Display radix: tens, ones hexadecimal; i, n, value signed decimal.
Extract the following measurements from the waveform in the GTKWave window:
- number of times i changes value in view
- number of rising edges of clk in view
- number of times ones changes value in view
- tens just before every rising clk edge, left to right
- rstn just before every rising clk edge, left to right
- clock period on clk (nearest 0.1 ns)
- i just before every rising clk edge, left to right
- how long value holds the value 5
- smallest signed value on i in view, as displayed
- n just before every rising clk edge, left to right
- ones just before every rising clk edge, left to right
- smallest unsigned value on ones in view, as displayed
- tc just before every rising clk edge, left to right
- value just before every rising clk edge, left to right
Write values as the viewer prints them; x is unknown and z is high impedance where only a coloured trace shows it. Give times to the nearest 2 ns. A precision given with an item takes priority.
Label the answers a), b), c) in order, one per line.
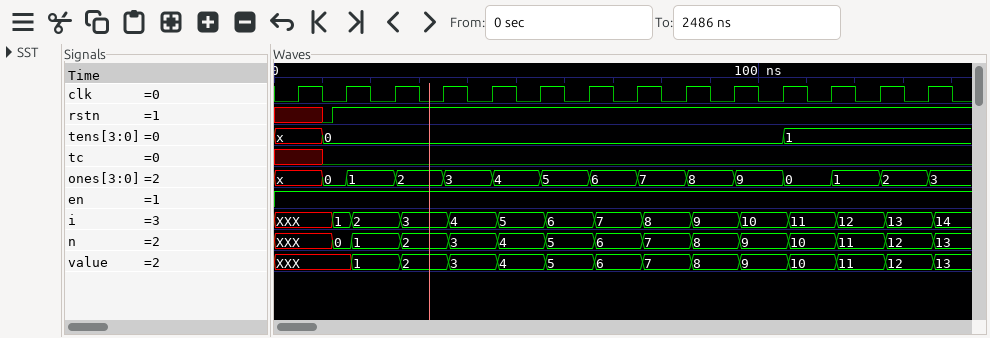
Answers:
a) 14
b) 14
c) 14
d) x, 0, 0, 0, 0, 0, 0, 0, 0, 0, 0, 1, 1, 1
e) x 1 1 1 1 1 1 1 1 1 1 1 1 1
f) 10 ns
g) XXX, 1, 2, 3, 4, 5, 6, 7, 8, 9, 10, 11, 12, 13
h) 10 ns
i) 1
j) XXX, 0, 1, 2, 3, 4, 5, 6, 7, 8, 9, 10, 11, 12
k) x, 0, 1, 2, 3, 4, 5, 6, 7, 8, 9, 0, 1, 2
l) 0
m) x 0 0 0 0 0 0 0 0 0 0 0 0 0
n) XXX, XXX, 1, 2, 3, 4, 5, 6, 7, 8, 9, 10, 11, 12
